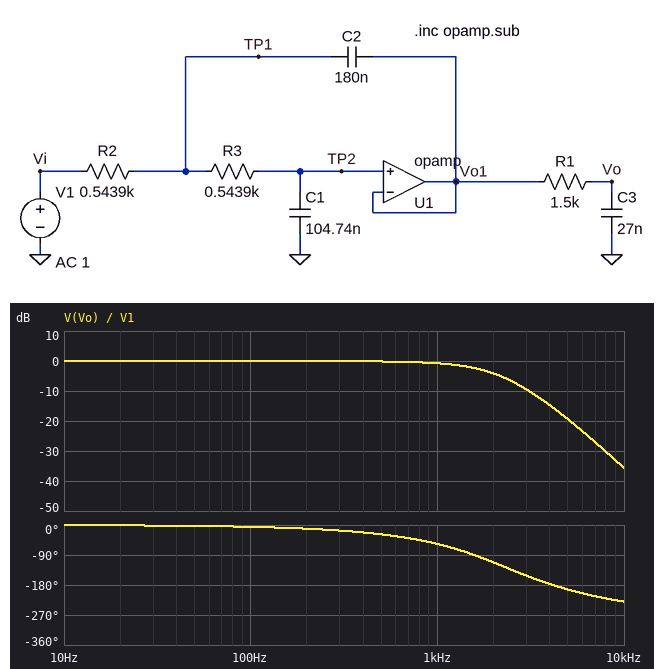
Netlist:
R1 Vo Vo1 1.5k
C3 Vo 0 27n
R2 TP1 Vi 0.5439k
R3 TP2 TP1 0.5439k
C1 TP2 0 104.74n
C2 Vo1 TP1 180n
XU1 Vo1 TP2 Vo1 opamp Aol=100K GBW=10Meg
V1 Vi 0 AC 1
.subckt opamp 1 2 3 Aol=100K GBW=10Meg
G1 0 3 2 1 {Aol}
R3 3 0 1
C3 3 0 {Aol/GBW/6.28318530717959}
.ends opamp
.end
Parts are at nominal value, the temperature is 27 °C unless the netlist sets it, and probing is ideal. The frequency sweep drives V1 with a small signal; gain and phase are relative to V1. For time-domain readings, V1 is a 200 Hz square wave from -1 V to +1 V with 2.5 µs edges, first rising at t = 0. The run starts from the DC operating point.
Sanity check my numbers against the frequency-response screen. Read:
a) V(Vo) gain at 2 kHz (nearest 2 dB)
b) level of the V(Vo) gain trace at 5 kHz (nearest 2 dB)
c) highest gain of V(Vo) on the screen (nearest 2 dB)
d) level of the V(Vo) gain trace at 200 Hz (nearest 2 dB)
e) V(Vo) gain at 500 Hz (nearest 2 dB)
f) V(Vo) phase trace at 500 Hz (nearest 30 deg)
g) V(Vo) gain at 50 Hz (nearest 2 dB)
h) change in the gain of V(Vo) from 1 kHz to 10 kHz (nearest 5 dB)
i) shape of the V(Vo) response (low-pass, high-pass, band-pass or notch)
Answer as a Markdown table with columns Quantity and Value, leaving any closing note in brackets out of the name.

| Quantity | Value |
|---|---|
| V(Vo) gain at 2 kHz | -4 dB |
| level of the V(Vo) gain trace at 5 kHz | -20 dB |
| highest gain of V(Vo) on the screen | 0 dB |
| level of the V(Vo) gain trace at 200 Hz | 0 dB |
| V(Vo) gain at 500 Hz | 0 dB |
| V(Vo) phase trace at 500 Hz | -30 deg |
| V(Vo) gain at 50 Hz | 0 dB |
| change in the gain of V(Vo) from 1 kHz to 10 kHz | -35 dB |
| shape of the V(Vo) response | low-pass |
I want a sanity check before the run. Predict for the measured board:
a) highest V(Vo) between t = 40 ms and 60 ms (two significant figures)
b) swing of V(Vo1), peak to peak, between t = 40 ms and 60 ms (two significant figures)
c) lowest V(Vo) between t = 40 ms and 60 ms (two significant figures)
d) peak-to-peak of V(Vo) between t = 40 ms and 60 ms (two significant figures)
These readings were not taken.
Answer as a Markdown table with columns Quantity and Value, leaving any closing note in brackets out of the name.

| Quantity | Value |
|---|---|
| highest V(Vo) between t = 40 ms and 60 ms | 1.0 V |
| swing of V(Vo1), peak to peak, between t = 40 ms and 60 ms | 2.1 V |
| lowest V(Vo) between t = 40 ms and 60 ms | -1.0 V |
| peak-to-peak of V(Vo) between t = 40 ms and 60 ms | 2.1 V |
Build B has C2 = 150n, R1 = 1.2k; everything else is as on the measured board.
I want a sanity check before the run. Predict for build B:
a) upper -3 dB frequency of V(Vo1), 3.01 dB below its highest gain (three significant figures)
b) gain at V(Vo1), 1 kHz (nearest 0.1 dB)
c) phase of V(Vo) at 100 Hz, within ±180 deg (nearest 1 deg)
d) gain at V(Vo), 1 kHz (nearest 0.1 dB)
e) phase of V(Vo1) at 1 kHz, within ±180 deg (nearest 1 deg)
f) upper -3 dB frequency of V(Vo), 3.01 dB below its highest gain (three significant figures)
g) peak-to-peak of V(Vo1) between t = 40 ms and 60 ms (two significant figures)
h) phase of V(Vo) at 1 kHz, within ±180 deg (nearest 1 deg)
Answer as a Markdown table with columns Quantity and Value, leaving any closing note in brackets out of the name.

| Quantity | Value |
|---|---|
| upper -3 dB frequency of V(Vo1), 3.01 dB below its highest gain | 1.92 kHz |
| gain at V(Vo1), 1 kHz | -0.7 dB |
| phase of V(Vo) at 100 Hz, within ±180 deg | -5 deg |
| gain at V(Vo), 1 kHz | -0.9 dB |
| phase of V(Vo1) at 1 kHz, within ±180 deg | -41 deg |
| upper -3 dB frequency of V(Vo), 3.01 dB below its highest gain | 1.76 kHz |
| peak-to-peak of V(Vo1) between t = 40 ms and 60 ms | 2.0 V |
| phase of V(Vo) at 1 kHz, within ±180 deg | -53 deg |
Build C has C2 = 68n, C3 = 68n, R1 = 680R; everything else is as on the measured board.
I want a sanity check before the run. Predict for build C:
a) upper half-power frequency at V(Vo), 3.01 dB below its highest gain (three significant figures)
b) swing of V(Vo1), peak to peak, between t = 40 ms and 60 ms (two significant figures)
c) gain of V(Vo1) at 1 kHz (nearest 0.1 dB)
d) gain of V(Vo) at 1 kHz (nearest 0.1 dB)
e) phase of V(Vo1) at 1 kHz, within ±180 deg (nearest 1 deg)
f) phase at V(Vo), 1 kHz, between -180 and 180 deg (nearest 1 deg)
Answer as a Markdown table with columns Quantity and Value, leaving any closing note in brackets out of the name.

| Quantity | Value |
|---|---|
| upper half-power frequency at V(Vo), 3.01 dB below its highest gain | 1.41 kHz |
| swing of V(Vo1), peak to peak, between t = 40 ms and 60 ms | 2.0 V |
| gain of V(Vo1) at 1 kHz | -1.3 dB |
| gain of V(Vo) at 1 kHz | -1.7 dB |
| phase of V(Vo1) at 1 kHz, within ±180 deg | -38 deg |
| phase at V(Vo), 1 kHz, between -180 and 180 deg | -54 deg |
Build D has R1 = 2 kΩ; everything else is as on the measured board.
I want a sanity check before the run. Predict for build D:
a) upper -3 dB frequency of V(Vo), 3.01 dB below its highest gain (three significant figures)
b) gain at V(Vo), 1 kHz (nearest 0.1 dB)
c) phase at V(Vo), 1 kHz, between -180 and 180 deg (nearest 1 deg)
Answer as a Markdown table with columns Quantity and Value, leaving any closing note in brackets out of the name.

| Quantity | Value |
|---|---|
| upper -3 dB frequency of V(Vo), 3.01 dB below its highest gain | 1.63 kHz |
| gain at V(Vo), 1 kHz | -1.0 dB |
| phase at V(Vo), 1 kHz, between -180 and 180 deg | -61 deg |
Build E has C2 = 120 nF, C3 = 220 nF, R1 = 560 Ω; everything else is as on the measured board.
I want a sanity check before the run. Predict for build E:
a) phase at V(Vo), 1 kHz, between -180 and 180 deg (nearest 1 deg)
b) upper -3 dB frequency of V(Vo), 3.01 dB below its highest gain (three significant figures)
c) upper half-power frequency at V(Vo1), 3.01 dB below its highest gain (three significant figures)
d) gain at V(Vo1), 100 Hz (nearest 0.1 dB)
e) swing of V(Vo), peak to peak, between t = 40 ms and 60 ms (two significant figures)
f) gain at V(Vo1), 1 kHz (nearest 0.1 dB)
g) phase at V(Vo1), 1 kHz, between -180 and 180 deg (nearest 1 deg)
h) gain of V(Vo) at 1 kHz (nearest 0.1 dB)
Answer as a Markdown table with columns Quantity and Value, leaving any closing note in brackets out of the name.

| Quantity | Value |
|---|---|
| phase at V(Vo), 1 kHz, between -180 and 180 deg | -78 deg |
| upper -3 dB frequency of V(Vo), 3.01 dB below its highest gain | 1.01 kHz |
| upper half-power frequency at V(Vo1), 3.01 dB below its highest gain | 1.85 kHz |
| gain at V(Vo1), 100 Hz | 0 dB |
| swing of V(Vo), peak to peak, between t = 40 ms and 60 ms | 2.0 V |
| gain at V(Vo1), 1 kHz | -0.9 dB |
| phase at V(Vo1), 1 kHz, between -180 and 180 deg | -40 deg |
| gain of V(Vo) at 1 kHz | -3.0 dB |
